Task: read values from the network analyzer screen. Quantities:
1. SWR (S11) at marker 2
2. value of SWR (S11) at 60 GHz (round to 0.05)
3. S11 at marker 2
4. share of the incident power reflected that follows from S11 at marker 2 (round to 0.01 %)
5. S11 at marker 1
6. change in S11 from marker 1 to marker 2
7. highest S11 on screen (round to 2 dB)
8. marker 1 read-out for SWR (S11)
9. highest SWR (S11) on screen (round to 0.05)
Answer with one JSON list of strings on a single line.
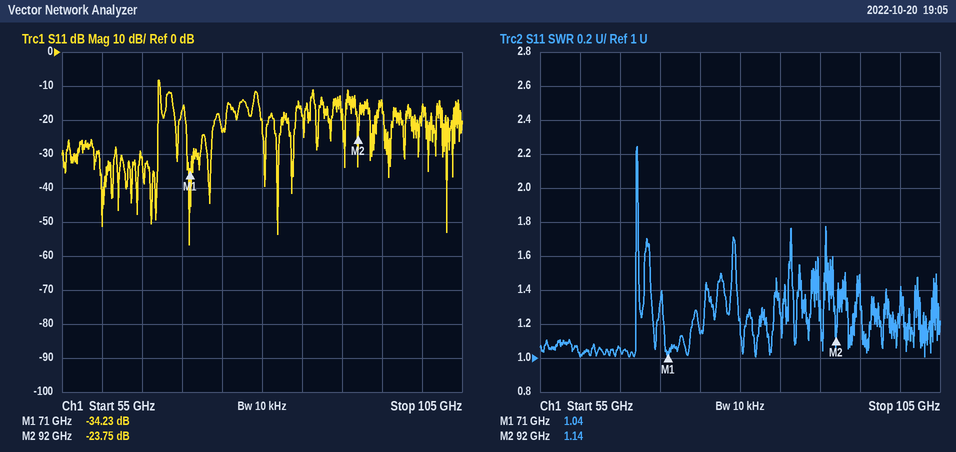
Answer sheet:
["1.14", "1.00", "-23.75 dB", "0.42 %", "-34.23 dB", "10.48 dB", "-8 dB", "1.04", "2.25"]
